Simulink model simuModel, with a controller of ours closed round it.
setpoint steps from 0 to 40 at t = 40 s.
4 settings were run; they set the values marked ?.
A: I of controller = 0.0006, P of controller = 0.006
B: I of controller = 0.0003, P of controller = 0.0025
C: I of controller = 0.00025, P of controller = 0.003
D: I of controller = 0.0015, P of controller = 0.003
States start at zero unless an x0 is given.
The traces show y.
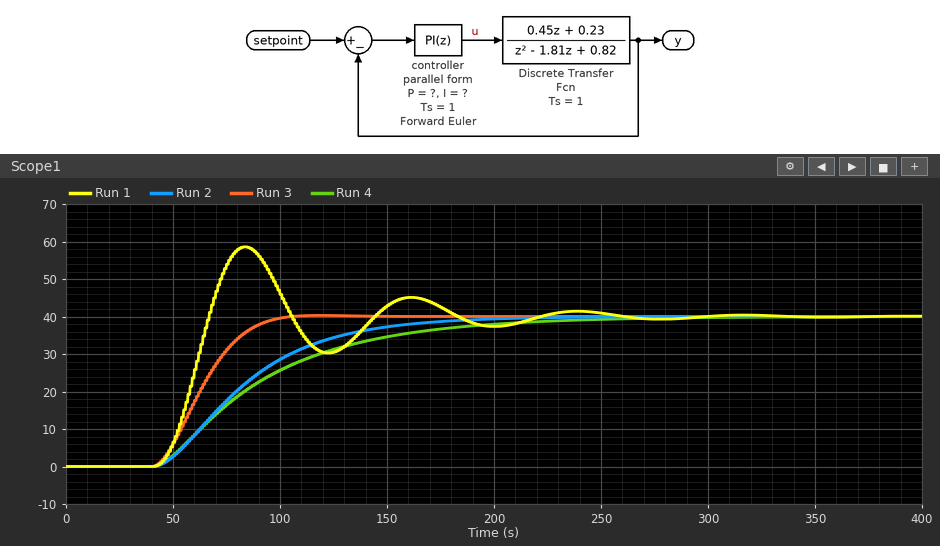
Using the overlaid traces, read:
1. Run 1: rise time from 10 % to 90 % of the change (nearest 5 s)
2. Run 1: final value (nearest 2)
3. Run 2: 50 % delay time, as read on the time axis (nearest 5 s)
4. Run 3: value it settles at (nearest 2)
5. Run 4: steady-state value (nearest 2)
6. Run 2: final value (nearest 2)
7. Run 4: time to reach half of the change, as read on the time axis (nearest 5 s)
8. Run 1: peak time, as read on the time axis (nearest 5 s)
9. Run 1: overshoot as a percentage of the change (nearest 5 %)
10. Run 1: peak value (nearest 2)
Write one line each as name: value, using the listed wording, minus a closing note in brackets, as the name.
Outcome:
Run 1: rise time from 10 % to 90 % of the change: 15 s
Run 1: final value: 40
Run 2: 50 % delay time, as read on the time axis: 80 s
Run 3: value it settles at: 40
Run 4: steady-state value: 40
Run 2: final value: 40
Run 4: time to reach half of the change, as read on the time axis: 85 s
Run 1: peak time, as read on the time axis: 85 s
Run 1: overshoot as a percentage of the change: 45 %
Run 1: peak value: 58
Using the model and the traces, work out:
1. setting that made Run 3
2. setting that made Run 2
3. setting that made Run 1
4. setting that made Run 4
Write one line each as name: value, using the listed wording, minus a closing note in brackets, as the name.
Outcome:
setting that made Run 3: A
setting that made Run 2: B
setting that made Run 1: D
setting that made Run 4: C
